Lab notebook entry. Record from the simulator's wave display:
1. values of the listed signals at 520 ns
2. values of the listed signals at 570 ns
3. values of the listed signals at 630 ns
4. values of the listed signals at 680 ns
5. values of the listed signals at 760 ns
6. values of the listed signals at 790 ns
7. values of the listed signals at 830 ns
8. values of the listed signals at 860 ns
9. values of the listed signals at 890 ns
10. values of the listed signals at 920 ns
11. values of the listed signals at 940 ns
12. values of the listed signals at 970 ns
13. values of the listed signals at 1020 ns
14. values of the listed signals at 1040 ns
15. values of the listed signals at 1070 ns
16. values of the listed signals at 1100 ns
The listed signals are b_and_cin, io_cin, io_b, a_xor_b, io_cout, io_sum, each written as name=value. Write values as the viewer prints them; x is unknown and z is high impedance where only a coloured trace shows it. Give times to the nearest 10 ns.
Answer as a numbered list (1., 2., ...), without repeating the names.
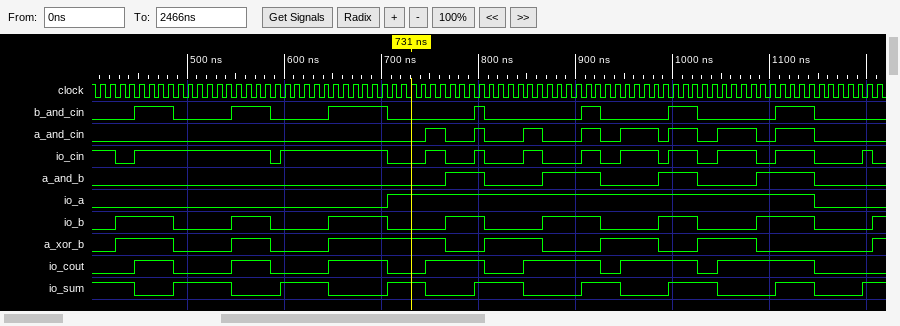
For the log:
1. b_and_cin=0, io_cin=1, io_b=0, a_xor_b=0, io_cout=0, io_sum=1
2. b_and_cin=1, io_cin=1, io_b=1, a_xor_b=1, io_cout=1, io_sum=0
3. b_and_cin=0, io_cin=1, io_b=0, a_xor_b=0, io_cout=0, io_sum=1
4. b_and_cin=1, io_cin=1, io_b=1, a_xor_b=1, io_cout=1, io_sum=0
5. b_and_cin=0, io_cin=1, io_b=0, a_xor_b=1, io_cout=1, io_sum=0
6. b_and_cin=0, io_cin=0, io_b=1, a_xor_b=0, io_cout=1, io_sum=0
7. b_and_cin=0, io_cin=0, io_b=0, a_xor_b=1, io_cout=0, io_sum=1
8. b_and_cin=0, io_cin=1, io_b=0, a_xor_b=1, io_cout=1, io_sum=0
9. b_and_cin=0, io_cin=0, io_b=1, a_xor_b=0, io_cout=1, io_sum=0
10. b_and_cin=1, io_cin=1, io_b=1, a_xor_b=0, io_cout=1, io_sum=1
11. b_and_cin=0, io_cin=0, io_b=0, a_xor_b=1, io_cout=0, io_sum=1
12. b_and_cin=0, io_cin=1, io_b=0, a_xor_b=1, io_cout=1, io_sum=0
13. b_and_cin=1, io_cin=1, io_b=1, a_xor_b=0, io_cout=1, io_sum=1
14. b_and_cin=0, io_cin=0, io_b=0, a_xor_b=1, io_cout=0, io_sum=1
15. b_and_cin=0, io_cin=1, io_b=0, a_xor_b=1, io_cout=1, io_sum=0
16. b_and_cin=0, io_cin=0, io_b=1, a_xor_b=0, io_cout=1, io_sum=0
